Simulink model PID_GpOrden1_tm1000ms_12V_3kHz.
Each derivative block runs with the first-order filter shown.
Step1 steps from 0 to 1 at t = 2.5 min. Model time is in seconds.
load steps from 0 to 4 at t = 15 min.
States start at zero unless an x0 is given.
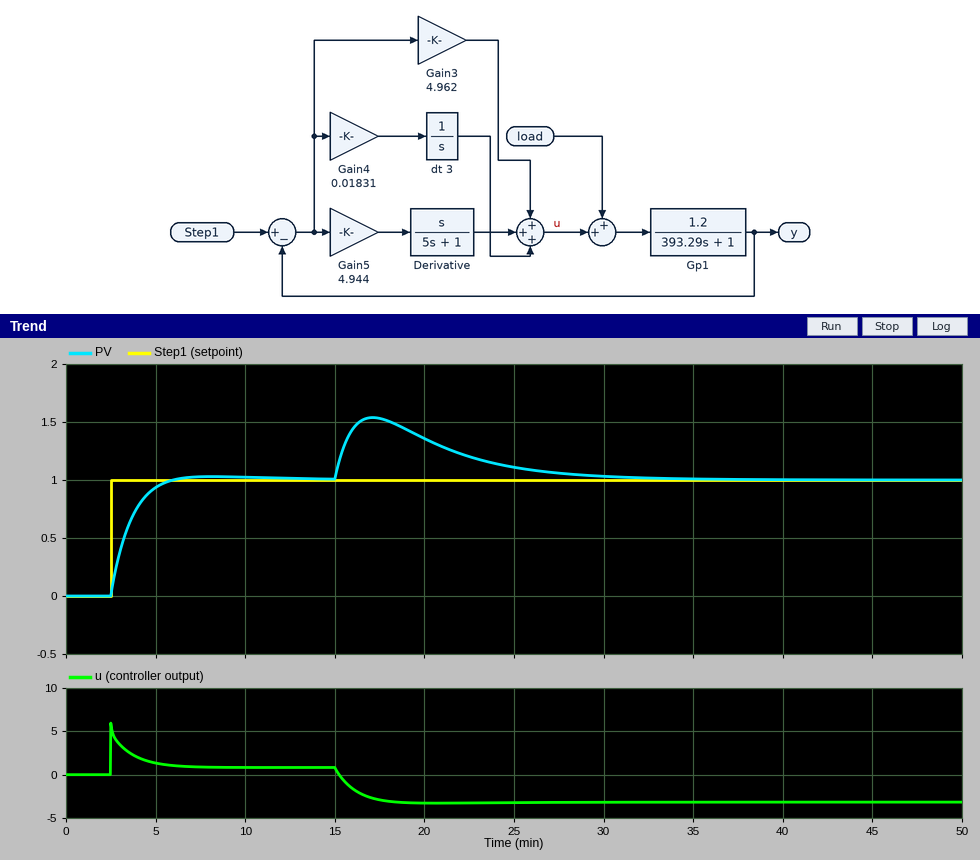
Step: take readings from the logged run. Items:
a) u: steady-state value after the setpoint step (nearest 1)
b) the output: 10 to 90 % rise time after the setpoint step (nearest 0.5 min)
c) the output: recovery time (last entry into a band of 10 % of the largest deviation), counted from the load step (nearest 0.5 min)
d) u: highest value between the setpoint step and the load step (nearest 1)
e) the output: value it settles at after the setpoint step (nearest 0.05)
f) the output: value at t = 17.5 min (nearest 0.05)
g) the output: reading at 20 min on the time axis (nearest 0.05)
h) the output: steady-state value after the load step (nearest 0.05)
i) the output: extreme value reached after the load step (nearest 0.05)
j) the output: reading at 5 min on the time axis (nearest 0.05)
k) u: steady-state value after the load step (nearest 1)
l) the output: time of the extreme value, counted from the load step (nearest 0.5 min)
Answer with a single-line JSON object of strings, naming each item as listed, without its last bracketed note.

{"u: steady-state value after the setpoint step": "1", "the output: 10 to 90 % rise time after the setpoint step": "2.0 min", "the output: recovery time (last entry into a band of 10 % of the largest deviation), counted from the load step": "13.0 min", "u: highest value between the setpoint step and the load step": "6", "the output: value it settles at after the setpoint step": "1.00", "the output: value at t = 17.5 min": "1.55", "the output: reading at 20 min on the time axis": "1.35", "the output: steady-state value after the load step": "1.00", "the output: extreme value reached after the load step": "1.55", "the output: reading at 5 min on the time axis": "0.95", "u: steady-state value after the load step": "-3", "the output: time of the extreme value, counted from the load step": "2.0 min"}
